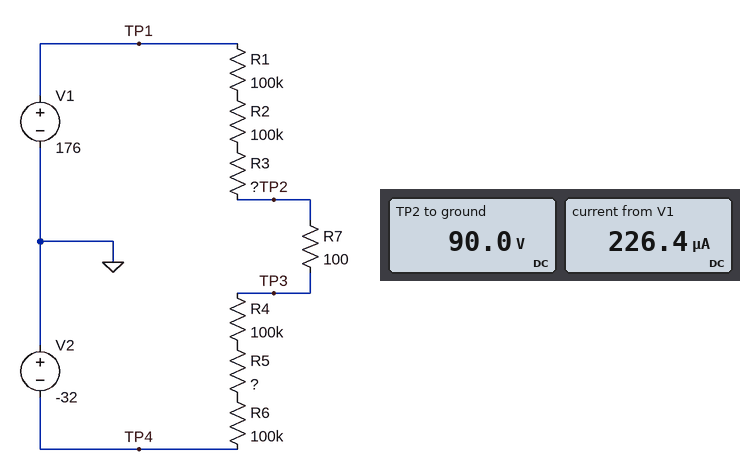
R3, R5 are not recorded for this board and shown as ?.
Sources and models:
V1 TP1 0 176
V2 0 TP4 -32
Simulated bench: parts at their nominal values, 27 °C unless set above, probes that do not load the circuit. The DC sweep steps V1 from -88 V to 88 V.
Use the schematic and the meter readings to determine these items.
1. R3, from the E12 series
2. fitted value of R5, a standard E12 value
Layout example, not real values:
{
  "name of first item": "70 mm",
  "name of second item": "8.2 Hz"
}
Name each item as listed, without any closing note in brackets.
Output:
{
  "R3, from the E12 series": "180 kΩ",
  "fitted value of R5, a standard E12 value": "56 kΩ"
}
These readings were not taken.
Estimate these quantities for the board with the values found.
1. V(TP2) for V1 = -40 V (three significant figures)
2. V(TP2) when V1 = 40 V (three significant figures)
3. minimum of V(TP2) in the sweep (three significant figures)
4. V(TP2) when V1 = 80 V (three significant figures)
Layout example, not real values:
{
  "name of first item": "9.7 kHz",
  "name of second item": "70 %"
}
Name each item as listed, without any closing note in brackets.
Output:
{
  "V(TP2) for V1 = -40 V": "3.01 V",
  "V(TP2) when V1 = 40 V": "35.2 V",
  "minimum of V(TP2) in the sweep": "-16.3 V",
  "V(TP2) when V1 = 80 V": "51.3 V"
}
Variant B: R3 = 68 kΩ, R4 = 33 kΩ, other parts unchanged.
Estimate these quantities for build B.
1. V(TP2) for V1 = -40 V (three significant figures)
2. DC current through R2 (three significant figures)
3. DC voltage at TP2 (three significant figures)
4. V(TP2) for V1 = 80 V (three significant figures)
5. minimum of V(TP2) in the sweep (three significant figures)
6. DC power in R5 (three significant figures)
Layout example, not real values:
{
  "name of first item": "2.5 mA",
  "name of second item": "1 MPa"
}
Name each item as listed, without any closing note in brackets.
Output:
{
  "V(TP2) for V1 = -40 V": "2.21 V",
  "DC current through R2": "315 µA",
  "DC voltage at TP2": "91.6 V",
  "V(TP2) for V1 = 80 V": "51.9 V",
  "minimum of V(TP2) in the sweep": "-17.6 V",
  "DC power in R5": "5.56 mW"
}
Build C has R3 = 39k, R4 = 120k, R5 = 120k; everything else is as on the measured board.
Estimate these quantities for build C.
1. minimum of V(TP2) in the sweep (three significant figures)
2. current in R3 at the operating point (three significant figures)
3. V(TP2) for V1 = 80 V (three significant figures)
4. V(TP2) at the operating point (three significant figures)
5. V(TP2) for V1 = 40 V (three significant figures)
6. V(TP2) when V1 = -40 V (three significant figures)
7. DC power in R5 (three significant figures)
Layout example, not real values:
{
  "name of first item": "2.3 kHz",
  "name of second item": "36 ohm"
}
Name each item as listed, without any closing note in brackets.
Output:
{
  "minimum of V(TP2) in the sweep": "-38.5 V",
  "current in R3 at the operating point": "249 µA",
  "V(TP2) for V1 = 80 V": "60.2 V",
  "V(TP2) at the operating point": "117 V",
  "V(TP2) for V1 = 40 V": "36.7 V",
  "V(TP2) when V1 = -40 V": "-10.3 V",
  "DC power in R5": "7.42 mW"
}
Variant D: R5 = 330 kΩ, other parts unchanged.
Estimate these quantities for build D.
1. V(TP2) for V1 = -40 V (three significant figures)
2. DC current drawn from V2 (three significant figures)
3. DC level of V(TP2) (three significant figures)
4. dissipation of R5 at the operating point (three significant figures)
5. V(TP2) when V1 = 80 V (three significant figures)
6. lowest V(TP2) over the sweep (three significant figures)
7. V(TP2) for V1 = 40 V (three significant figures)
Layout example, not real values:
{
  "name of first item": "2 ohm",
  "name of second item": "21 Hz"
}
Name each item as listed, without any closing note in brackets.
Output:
{
  "V(TP2) for V1 = -40 V": "-9.94 V",
  "DC current drawn from V2": "158 µA",
  "DC level of V(TP2)": "116 V",
  "dissipation of R5 at the operating point": "8.26 mW",
  "V(TP2) when V1 = 80 V": "60.0 V",
  "lowest V(TP2) over the sweep": "-37.9 V",
  "V(TP2) for V1 = 40 V": "36.7 V"
}
